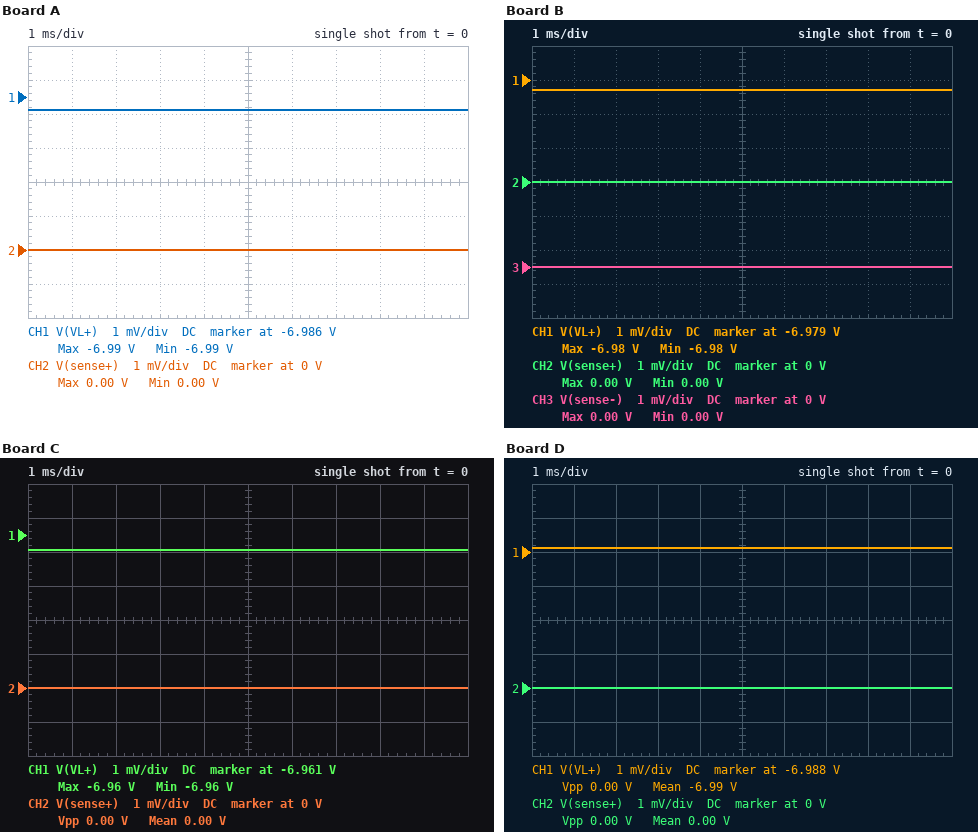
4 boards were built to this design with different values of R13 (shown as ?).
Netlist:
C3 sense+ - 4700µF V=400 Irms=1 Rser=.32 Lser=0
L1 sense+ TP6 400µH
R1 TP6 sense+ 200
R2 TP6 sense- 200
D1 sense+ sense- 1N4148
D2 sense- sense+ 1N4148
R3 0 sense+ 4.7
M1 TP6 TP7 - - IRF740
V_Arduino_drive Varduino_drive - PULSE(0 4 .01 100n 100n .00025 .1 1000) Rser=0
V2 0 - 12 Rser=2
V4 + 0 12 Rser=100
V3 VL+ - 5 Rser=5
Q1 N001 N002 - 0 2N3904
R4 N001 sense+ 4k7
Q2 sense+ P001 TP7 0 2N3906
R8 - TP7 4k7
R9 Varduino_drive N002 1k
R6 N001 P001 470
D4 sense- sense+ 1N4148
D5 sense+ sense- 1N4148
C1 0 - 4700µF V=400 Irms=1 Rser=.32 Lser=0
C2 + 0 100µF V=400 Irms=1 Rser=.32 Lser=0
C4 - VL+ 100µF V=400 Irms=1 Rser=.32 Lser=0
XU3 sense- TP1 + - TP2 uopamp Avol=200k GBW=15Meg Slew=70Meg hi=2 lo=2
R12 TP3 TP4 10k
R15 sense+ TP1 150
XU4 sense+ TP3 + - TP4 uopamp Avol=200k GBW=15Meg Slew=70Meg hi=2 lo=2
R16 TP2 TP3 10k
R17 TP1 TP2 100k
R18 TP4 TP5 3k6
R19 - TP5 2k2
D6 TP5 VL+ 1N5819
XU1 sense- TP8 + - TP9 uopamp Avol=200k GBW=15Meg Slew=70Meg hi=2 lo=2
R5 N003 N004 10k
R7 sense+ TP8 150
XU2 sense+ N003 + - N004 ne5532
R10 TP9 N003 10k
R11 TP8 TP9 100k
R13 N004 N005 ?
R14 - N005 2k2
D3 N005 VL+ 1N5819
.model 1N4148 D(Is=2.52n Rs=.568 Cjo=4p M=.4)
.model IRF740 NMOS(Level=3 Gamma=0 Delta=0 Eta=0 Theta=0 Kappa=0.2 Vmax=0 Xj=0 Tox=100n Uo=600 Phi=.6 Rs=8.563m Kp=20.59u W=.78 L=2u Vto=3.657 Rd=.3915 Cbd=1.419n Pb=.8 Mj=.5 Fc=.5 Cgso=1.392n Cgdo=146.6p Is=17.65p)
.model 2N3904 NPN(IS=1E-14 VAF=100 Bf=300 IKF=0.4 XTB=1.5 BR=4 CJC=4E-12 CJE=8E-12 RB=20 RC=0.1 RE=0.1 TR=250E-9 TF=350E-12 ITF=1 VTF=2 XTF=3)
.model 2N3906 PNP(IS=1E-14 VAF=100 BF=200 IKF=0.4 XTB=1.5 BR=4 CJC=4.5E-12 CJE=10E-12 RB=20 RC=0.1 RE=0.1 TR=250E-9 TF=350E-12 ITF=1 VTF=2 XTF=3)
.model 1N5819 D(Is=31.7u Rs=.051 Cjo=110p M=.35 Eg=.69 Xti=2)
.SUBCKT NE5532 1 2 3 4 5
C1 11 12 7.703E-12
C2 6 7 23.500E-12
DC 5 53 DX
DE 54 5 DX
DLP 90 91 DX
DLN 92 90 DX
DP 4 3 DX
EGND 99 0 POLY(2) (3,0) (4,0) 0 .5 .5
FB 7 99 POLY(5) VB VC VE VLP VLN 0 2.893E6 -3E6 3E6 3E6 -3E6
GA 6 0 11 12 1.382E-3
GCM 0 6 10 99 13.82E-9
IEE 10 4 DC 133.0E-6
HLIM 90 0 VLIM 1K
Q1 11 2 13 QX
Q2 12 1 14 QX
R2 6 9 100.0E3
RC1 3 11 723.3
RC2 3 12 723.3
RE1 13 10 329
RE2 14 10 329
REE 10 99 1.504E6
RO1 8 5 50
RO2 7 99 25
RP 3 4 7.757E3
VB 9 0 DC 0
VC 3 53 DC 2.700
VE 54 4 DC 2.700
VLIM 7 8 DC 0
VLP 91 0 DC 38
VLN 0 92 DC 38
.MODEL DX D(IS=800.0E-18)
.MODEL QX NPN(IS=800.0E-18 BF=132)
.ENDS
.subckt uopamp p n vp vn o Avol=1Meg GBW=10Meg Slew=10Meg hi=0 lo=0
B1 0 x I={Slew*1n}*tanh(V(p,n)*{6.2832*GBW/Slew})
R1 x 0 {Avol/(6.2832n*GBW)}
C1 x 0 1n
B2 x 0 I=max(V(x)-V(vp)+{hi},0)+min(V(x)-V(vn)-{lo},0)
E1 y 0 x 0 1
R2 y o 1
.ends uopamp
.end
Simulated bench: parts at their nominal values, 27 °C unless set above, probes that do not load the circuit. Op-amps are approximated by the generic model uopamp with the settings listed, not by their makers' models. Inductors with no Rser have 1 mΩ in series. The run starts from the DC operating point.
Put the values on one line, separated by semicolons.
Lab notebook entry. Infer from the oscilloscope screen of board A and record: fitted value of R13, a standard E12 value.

4.7 kΩ
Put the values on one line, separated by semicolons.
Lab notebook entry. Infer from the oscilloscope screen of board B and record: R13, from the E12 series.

2.2 kΩ
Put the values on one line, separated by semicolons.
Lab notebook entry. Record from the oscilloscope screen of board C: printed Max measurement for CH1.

-6.96 V
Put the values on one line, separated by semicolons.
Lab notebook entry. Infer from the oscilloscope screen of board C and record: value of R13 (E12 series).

1.2 kΩ
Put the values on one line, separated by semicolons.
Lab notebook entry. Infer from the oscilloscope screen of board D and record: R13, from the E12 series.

10 kΩ
